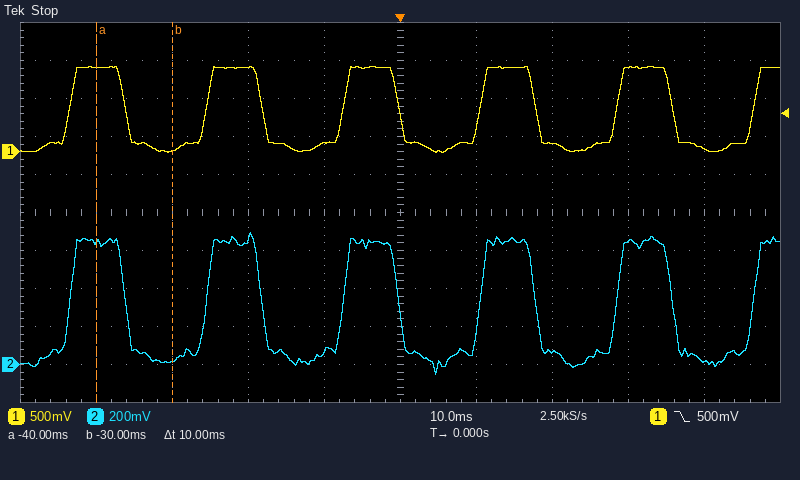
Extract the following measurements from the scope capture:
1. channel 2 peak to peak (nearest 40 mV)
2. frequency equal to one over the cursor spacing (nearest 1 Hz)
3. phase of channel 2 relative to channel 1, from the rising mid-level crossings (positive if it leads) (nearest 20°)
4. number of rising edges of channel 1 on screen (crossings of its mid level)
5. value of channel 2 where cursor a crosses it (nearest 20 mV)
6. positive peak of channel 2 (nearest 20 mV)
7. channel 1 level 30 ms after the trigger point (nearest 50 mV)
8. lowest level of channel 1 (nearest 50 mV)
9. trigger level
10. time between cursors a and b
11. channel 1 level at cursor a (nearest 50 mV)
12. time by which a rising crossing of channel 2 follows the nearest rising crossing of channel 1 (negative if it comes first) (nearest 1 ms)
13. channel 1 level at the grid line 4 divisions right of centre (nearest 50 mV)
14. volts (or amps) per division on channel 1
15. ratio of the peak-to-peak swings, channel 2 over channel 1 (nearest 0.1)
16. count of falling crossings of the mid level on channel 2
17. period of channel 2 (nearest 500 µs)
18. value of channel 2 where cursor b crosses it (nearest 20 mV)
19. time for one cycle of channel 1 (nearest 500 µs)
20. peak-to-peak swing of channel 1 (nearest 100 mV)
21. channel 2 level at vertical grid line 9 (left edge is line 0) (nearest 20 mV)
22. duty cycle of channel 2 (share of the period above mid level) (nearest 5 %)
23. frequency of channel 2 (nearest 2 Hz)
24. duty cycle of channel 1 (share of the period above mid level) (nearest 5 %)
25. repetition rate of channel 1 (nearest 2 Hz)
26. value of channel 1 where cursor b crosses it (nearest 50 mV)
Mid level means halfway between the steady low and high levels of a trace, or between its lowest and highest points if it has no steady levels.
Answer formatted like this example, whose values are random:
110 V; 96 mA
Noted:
760 mV; 100 Hz; 0°; 6; 640 mV; 700 mV; 1.10 V; 0 mV; 500 mV; 10 ms; 1.10 V; 0 ms; 50 mV; 500 mV; 0.7; 5; 18.0 ms; 20 mV; 18.0 ms; 1.10 V; 20 mV; 40 %; 56 Hz; 40 %; 56 Hz; 0 mV
